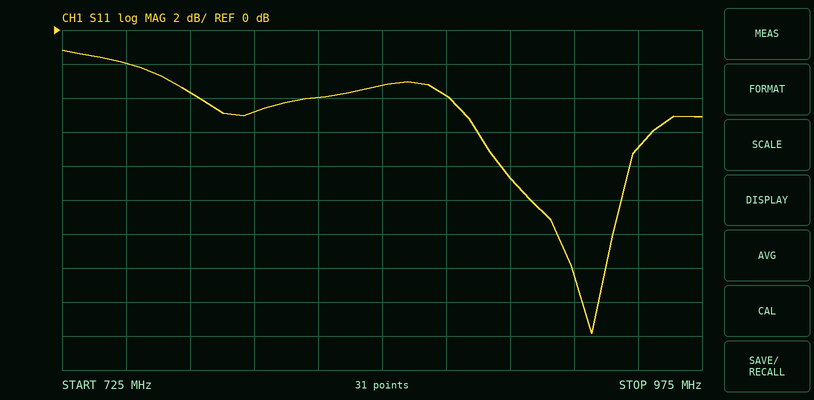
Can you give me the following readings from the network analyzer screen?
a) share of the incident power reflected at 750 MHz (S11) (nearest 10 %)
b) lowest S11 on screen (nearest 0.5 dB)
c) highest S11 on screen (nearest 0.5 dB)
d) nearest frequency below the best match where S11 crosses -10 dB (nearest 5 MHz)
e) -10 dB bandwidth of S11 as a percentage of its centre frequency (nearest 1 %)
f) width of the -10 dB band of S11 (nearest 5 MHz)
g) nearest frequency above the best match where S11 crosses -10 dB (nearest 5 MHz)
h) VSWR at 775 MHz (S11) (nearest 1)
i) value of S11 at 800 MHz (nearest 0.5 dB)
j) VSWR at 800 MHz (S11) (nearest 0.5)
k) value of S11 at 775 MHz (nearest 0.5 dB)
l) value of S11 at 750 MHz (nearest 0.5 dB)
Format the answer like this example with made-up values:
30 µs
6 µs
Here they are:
60 %
-18.0 dB
-1.0 dB
910 MHz
4 %
35 MHz
945 MHz
5
-5.0 dB
3.5
-3.5 dB
-2.0 dB
